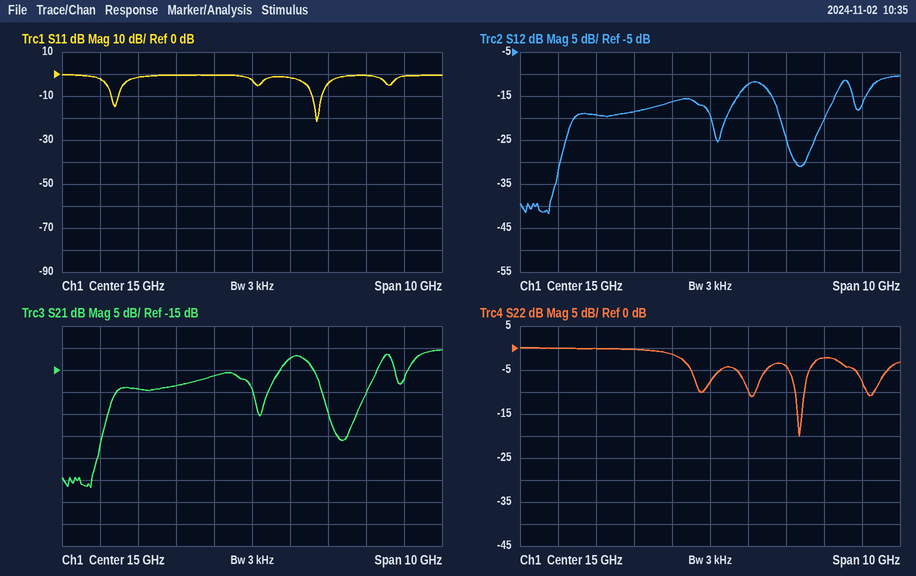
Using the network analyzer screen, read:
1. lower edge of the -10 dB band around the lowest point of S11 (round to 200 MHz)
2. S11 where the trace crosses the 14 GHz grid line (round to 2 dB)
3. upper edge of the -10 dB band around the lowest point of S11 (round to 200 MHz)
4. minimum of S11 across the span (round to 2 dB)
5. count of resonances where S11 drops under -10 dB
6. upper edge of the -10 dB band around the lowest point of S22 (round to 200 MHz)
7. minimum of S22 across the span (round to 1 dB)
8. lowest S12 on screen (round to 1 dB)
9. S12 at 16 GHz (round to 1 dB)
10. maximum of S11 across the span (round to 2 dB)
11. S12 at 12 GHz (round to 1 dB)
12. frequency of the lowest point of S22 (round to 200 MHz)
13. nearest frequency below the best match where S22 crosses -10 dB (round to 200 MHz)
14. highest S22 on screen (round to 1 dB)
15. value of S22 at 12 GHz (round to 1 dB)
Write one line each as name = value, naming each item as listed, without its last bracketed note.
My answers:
lower edge of the -10 dB band around the lowest point of S11 = 16.6 GHz
S11 where the trace crosses the 14 GHz grid line = 0 dB
upper edge of the -10 dB band around the lowest point of S11 = 16.8 GHz
minimum of S11 across the span = -22 dB
count of resonances where S11 drops under -10 dB = 2
upper edge of the -10 dB band around the lowest point of S22 = 17.4 GHz
minimum of S22 across the span = -20 dB
lowest S12 on screen = -42 dB
S12 at 16 GHz = -12 dB
maximum of S11 across the span = 0 dB
S12 at 12 GHz = -19 dB
frequency of the lowest point of S22 = 17.4 GHz
nearest frequency below the best match where S22 crosses -10 dB = 17.2 GHz
highest S22 on screen = 0 dB
value of S22 at 12 GHz = 0 dB
